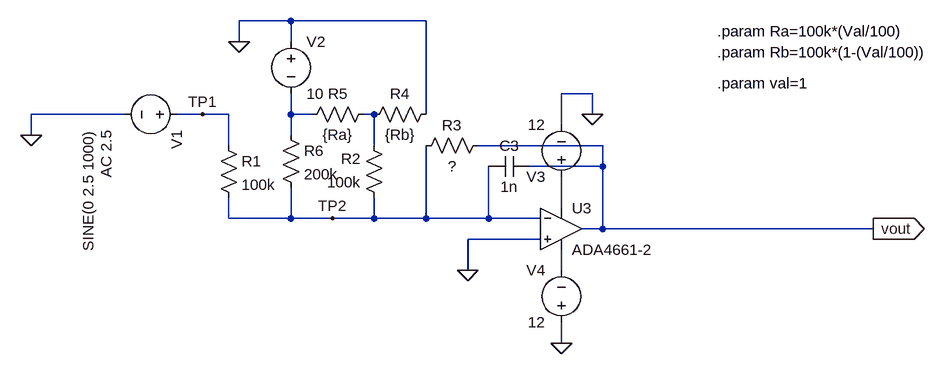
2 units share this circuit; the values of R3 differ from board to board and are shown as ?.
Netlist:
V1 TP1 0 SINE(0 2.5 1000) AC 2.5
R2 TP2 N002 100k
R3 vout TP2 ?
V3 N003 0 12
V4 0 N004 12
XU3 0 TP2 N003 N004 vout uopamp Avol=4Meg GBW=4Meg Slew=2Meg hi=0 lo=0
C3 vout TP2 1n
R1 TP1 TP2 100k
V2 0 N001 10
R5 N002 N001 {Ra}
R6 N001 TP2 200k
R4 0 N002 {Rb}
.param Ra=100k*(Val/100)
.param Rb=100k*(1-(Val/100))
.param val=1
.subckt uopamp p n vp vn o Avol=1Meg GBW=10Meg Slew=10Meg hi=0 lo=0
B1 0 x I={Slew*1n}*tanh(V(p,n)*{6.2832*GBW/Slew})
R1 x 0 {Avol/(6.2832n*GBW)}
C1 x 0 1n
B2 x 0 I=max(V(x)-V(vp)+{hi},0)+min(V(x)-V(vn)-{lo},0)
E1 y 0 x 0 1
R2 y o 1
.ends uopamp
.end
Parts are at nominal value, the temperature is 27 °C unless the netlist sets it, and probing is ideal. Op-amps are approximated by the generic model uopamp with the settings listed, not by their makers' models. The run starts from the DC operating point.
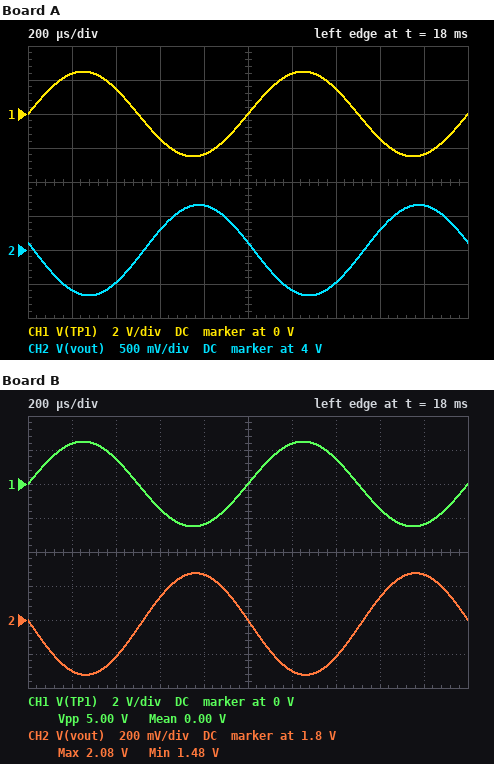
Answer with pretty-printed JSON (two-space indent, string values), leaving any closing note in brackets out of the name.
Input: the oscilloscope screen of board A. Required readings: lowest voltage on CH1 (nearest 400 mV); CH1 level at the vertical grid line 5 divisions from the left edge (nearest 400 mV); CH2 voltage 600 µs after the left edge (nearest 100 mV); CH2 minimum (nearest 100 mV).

{
  "lowest voltage on CH1": "-2.4 V",
  "CH1 level at the vertical grid line 5 divisions from the left edge": "0 V",
  "CH2 voltage 600 µs after the left edge": "4.3 V",
  "CH2 minimum": "3.3 V"
}
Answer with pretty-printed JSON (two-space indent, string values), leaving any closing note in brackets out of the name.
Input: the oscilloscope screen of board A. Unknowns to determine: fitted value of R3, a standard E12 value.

{
  "fitted value of R3, a standard E12 value": "27 kΩ"
}
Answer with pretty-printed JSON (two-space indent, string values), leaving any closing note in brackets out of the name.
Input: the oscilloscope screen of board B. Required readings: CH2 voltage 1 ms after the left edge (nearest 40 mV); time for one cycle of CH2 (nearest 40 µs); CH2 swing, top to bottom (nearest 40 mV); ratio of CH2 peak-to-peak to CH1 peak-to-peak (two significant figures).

{
  "CH2 voltage 1 ms after the left edge": "1.80 V",
  "time for one cycle of CH2": "1.00 ms",
  "CH2 swing, top to bottom": "600 mV",
  "ratio of CH2 peak-to-peak to CH1 peak-to-peak": "0.12"
}
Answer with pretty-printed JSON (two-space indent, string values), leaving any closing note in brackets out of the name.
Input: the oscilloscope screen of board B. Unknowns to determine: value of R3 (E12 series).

{
  "value of R3": "12 kΩ"
}
